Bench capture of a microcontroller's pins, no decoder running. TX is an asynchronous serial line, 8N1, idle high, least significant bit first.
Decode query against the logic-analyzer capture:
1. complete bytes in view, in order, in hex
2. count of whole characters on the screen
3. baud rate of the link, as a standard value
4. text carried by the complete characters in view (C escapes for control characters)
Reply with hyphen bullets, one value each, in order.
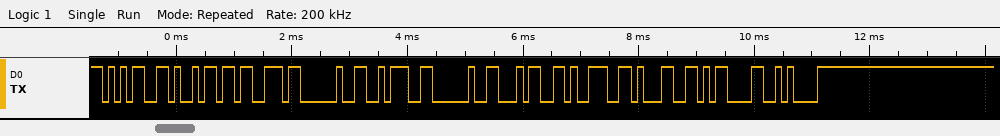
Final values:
- 0x35 0x69 0x73 0x20 0x3A 0x20 0x34 0x39 0x31 0x0D 0x0A
- 11
- 9600 baud
- "5is : 491\r\n"
